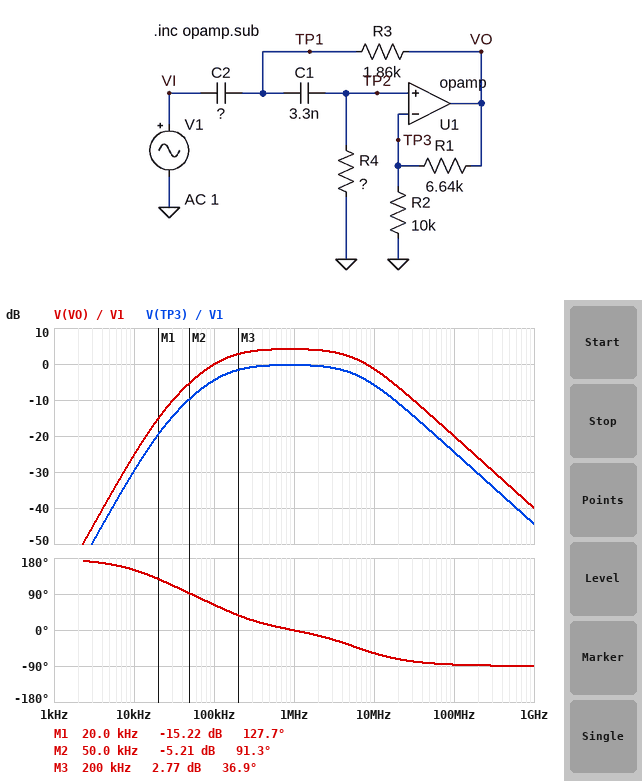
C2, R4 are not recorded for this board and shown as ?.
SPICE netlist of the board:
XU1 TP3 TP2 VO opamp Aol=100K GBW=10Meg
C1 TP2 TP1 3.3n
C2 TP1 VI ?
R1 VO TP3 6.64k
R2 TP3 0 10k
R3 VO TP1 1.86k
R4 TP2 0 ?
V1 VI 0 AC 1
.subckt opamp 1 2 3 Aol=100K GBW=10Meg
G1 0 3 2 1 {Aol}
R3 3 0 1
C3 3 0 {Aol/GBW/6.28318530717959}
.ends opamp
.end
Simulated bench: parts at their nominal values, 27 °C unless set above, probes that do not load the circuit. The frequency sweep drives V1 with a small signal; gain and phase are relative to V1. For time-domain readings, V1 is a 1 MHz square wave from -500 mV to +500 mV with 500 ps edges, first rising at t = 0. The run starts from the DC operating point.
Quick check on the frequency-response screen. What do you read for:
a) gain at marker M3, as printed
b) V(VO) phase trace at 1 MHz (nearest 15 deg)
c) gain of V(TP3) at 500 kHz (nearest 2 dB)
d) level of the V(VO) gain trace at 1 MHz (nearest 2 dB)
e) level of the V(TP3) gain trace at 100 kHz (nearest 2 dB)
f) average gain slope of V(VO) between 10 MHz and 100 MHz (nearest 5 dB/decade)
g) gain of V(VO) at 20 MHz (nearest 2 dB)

2.77 dB
0 deg
0 dB
4 dB
-4 dB
-20 dB/decade
-6 dB
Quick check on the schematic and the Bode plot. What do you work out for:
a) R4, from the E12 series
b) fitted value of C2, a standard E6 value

680 Ω
2.2 nF
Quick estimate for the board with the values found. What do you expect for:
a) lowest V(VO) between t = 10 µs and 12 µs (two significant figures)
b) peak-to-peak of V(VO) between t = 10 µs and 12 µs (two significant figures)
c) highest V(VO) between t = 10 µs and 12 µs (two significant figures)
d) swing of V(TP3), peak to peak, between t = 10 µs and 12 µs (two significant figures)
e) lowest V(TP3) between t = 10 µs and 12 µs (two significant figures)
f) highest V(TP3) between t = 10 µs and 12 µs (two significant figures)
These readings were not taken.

-950 mV
1.8 V
880 mV
1.1 V
-570 mV
530 mV
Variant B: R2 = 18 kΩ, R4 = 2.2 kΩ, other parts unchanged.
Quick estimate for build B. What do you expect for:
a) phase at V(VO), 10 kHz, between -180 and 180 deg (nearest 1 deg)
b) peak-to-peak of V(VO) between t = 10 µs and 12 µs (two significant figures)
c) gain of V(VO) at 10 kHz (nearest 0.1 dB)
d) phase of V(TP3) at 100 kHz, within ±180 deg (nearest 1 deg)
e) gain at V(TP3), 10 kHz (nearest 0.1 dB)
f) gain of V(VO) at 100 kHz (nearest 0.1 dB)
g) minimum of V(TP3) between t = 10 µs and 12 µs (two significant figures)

152 deg
1.4 V
-15.9 dB
23 deg
-18.6 dB
2.7 dB
-620 mV
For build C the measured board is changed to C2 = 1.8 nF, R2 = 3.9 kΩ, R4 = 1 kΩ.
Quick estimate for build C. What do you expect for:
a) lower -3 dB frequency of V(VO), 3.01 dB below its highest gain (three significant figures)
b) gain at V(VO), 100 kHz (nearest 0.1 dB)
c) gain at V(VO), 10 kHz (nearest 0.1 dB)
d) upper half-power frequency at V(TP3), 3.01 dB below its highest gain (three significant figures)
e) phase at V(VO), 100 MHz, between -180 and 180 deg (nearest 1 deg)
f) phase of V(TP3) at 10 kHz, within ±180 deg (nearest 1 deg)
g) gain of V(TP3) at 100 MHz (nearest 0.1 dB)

41.5 kHz
8.8 dB
-18.4 dB
3.34 MHz
-88 deg
166 deg
-28.6 dB
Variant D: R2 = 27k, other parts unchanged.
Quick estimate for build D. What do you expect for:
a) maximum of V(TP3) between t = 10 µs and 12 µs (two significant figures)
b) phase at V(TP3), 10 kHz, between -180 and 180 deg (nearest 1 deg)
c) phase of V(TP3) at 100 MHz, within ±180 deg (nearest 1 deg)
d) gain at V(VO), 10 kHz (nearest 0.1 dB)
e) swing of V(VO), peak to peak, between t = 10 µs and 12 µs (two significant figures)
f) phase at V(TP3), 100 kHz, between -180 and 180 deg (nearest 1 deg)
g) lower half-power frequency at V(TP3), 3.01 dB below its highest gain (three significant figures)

550 mV
148 deg
-85 deg
-28.0 dB
1.4 V
66 deg
145 kHz
